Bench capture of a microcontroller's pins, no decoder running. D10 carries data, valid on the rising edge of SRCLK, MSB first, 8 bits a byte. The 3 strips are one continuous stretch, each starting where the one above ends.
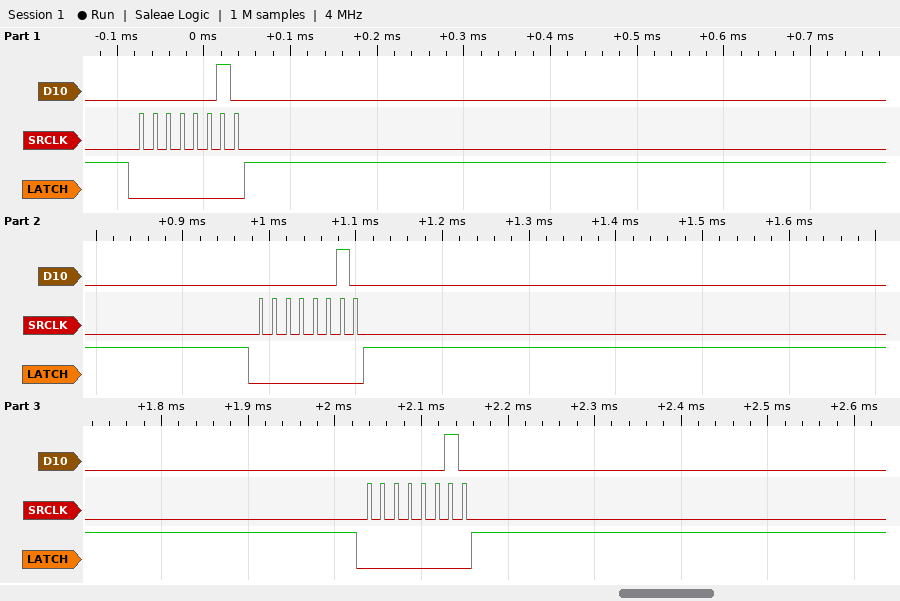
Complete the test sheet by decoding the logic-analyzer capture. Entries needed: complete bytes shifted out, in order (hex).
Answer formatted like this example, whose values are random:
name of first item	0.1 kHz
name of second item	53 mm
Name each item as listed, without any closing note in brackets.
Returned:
complete bytes shifted out, in order	02 02 02
